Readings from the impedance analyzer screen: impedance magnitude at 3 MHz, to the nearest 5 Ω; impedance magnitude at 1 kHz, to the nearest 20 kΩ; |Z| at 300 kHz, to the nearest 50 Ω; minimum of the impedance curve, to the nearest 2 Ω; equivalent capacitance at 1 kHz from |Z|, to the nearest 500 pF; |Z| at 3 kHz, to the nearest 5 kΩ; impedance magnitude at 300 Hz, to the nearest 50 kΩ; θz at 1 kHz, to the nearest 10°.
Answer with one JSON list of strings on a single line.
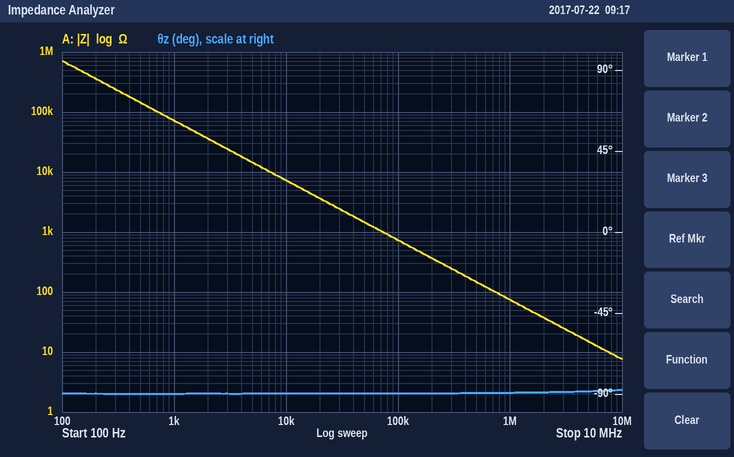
["25 Ω", "80 kΩ", "250 Ω", "8 Ω", "2.0 nF", "25 kΩ", "250 kΩ", "-90°"]
